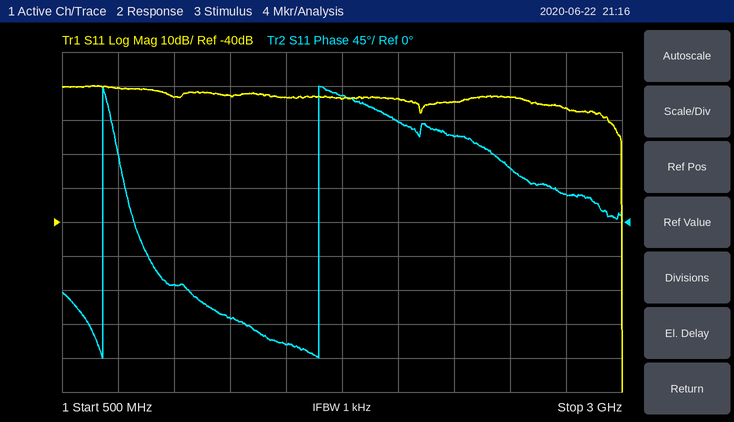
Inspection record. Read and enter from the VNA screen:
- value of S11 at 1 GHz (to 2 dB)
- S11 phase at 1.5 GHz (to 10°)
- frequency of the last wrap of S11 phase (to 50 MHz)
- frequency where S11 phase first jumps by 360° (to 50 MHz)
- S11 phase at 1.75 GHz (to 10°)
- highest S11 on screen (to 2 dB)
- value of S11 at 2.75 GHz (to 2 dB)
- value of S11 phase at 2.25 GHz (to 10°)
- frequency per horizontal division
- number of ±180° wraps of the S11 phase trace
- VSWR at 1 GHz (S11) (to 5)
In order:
-4 dB
-160°
1.65 GHz
700 MHz
170°
0 dB
-6 dB
110°
250 MHz
2
5
